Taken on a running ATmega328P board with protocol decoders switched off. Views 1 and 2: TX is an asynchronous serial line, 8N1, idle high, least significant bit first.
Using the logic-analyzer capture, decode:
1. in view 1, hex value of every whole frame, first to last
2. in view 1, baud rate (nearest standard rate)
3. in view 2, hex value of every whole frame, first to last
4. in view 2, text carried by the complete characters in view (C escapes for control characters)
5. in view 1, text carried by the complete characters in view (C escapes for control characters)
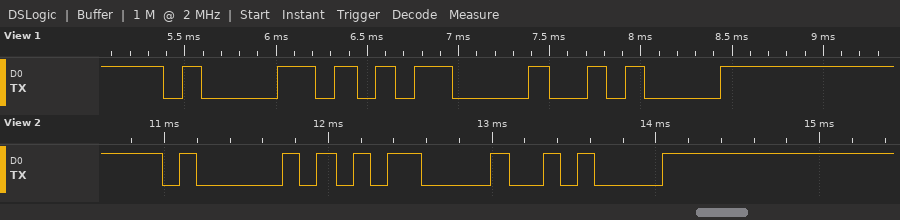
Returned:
0x61 0x0D 0x0A
9600 baud
0x41 0x0D 0x0A
"A\r\n"
"a\r\n"
